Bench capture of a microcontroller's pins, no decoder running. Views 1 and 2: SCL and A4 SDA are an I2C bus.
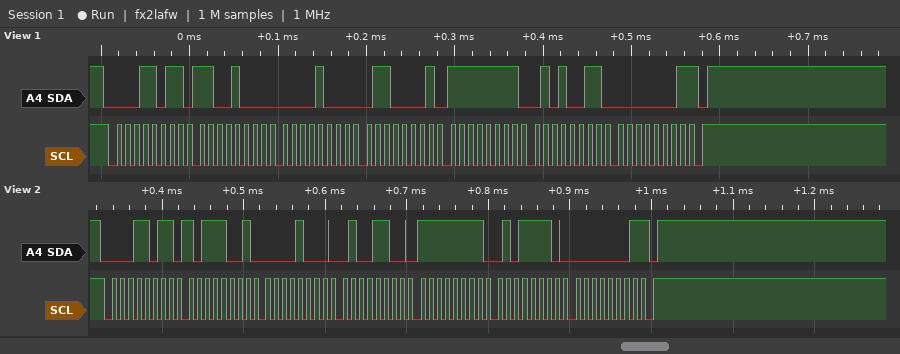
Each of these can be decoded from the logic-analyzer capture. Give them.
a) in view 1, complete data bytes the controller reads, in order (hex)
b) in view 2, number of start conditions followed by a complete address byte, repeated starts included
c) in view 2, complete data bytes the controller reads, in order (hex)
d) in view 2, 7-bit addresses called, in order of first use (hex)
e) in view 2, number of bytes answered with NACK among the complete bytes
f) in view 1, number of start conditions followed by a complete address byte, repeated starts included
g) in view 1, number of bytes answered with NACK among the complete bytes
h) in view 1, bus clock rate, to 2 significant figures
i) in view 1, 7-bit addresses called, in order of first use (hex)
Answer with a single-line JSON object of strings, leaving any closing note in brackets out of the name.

{"in view 1, complete data bytes the controller reads, in order": "C8 08 61 FF 53 01", "in view 2, number of start conditions followed by a complete address byte, repeated starts included": "1", "in view 2, complete data bytes the controller reads, in order": "B9 08 4C FF 5E 01", "in view 2, 7-bit addresses called, in order of first use": "0x0D", "in view 2, number of bytes answered with NACK among the complete bytes": "1", "in view 1, number of start conditions followed by a complete address byte, repeated starts included": "1", "in view 1, number of bytes answered with NACK among the complete bytes": "1", "in view 1, bus clock rate, to 2 significant figures": "100 kHz", "in view 1, 7-bit addresses called, in order of first use": "0x0D"}
